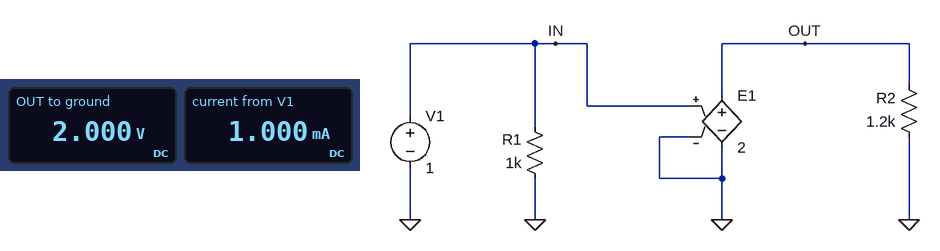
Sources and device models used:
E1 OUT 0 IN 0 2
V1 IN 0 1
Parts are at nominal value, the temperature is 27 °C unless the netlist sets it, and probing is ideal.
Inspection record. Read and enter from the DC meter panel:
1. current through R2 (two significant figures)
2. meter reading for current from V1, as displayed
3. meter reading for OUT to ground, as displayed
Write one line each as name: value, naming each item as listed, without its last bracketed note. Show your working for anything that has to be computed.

current through R2: (2 V) / 1.2 kΩ = 1.7 mA
meter reading for current from V1, as displayed: 1.000 mA
meter reading for OUT to ground, as displayed: 2.000 V
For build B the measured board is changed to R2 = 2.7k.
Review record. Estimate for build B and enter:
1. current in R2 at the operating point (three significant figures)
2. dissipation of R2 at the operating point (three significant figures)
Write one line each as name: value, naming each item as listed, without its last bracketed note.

current in R2 at the operating point: 741 µA
dissipation of R2 at the operating point: 1.48 mW
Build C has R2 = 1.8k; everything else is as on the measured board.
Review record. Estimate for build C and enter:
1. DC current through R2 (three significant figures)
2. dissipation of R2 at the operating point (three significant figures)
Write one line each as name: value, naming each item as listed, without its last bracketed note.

DC current through R2: 1.11 mA
dissipation of R2 at the operating point: 2.22 mW
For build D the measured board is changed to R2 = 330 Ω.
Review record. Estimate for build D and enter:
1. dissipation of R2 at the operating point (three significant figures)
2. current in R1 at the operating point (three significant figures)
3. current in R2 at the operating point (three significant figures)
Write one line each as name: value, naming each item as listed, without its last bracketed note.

dissipation of R2 at the operating point: 12.1 mW
current in R1 at the operating point: 1.00 mA
current in R2 at the operating point: 6.06 mA
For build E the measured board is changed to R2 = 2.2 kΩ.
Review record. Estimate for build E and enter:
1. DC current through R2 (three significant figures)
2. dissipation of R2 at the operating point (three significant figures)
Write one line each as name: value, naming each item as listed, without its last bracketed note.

DC current through R2: 909 µA
dissipation of R2 at the operating point: 1.82 mW
